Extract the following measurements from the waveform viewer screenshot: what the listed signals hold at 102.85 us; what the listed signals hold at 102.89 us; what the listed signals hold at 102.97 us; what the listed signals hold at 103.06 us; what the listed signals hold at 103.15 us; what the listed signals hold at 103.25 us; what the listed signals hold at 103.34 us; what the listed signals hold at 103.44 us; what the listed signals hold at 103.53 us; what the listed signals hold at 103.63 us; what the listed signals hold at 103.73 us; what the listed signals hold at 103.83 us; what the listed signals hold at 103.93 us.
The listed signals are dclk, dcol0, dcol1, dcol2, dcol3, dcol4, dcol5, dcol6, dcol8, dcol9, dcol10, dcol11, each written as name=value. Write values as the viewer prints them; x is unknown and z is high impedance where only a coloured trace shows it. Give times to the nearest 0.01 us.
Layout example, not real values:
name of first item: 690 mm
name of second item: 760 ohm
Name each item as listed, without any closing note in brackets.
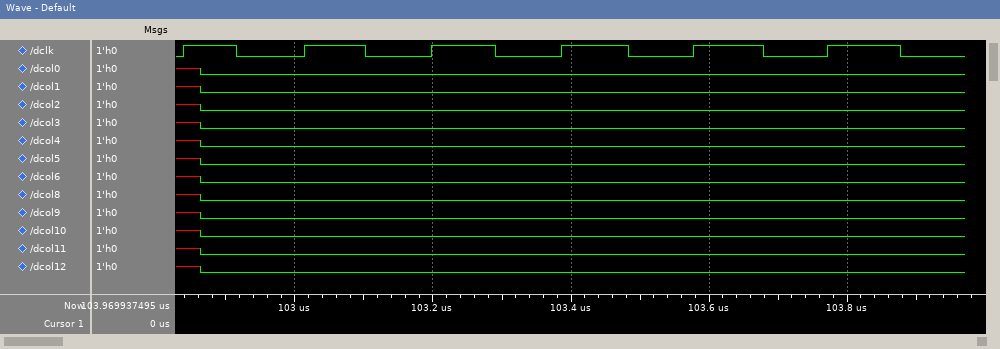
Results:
what the listed signals hold at 102.85 us: dclk=1, dcol0=x, dcol1=x, dcol2=x, dcol3=x, dcol4=x, dcol5=x, dcol6=x, dcol8=x, dcol9=x, dcol10=x, dcol11=x
what the listed signals hold at 102.89 us: dclk=1, dcol0=0, dcol1=0, dcol2=0, dcol3=0, dcol4=0, dcol5=0, dcol6=0, dcol8=0, dcol9=0, dcol10=0, dcol11=0
what the listed signals hold at 102.97 us: dclk=0, dcol0=0, dcol1=0, dcol2=0, dcol3=0, dcol4=0, dcol5=0, dcol6=0, dcol8=0, dcol9=0, dcol10=0, dcol11=0
what the listed signals hold at 103.06 us: dclk=1, dcol0=0, dcol1=0, dcol2=0, dcol3=0, dcol4=0, dcol5=0, dcol6=0, dcol8=0, dcol9=0, dcol10=0, dcol11=0
what the listed signals hold at 103.15 us: dclk=0, dcol0=0, dcol1=0, dcol2=0, dcol3=0, dcol4=0, dcol5=0, dcol6=0, dcol8=0, dcol9=0, dcol10=0, dcol11=0
what the listed signals hold at 103.25 us: dclk=1, dcol0=0, dcol1=0, dcol2=0, dcol3=0, dcol4=0, dcol5=0, dcol6=0, dcol8=0, dcol9=0, dcol10=0, dcol11=0
what the listed signals hold at 103.34 us: dclk=0, dcol0=0, dcol1=0, dcol2=0, dcol3=0, dcol4=0, dcol5=0, dcol6=0, dcol8=0, dcol9=0, dcol10=0, dcol11=0
what the listed signals hold at 103.44 us: dclk=1, dcol0=0, dcol1=0, dcol2=0, dcol3=0, dcol4=0, dcol5=0, dcol6=0, dcol8=0, dcol9=0, dcol10=0, dcol11=0
what the listed signals hold at 103.53 us: dclk=0, dcol0=0, dcol1=0, dcol2=0, dcol3=0, dcol4=0, dcol5=0, dcol6=0, dcol8=0, dcol9=0, dcol10=0, dcol11=0
what the listed signals hold at 103.63 us: dclk=1, dcol0=0, dcol1=0, dcol2=0, dcol3=0, dcol4=0, dcol5=0, dcol6=0, dcol8=0, dcol9=0, dcol10=0, dcol11=0
what the listed signals hold at 103.73 us: dclk=0, dcol0=0, dcol1=0, dcol2=0, dcol3=0, dcol4=0, dcol5=0, dcol6=0, dcol8=0, dcol9=0, dcol10=0, dcol11=0
what the listed signals hold at 103.83 us: dclk=1, dcol0=0, dcol1=0, dcol2=0, dcol3=0, dcol4=0, dcol5=0, dcol6=0, dcol8=0, dcol9=0, dcol10=0, dcol11=0
what the listed signals hold at 103.93 us: dclk=0, dcol0=0, dcol1=0, dcol2=0, dcol3=0, dcol4=0, dcol5=0, dcol6=0, dcol8=0, dcol9=0, dcol10=0, dcol11=0
